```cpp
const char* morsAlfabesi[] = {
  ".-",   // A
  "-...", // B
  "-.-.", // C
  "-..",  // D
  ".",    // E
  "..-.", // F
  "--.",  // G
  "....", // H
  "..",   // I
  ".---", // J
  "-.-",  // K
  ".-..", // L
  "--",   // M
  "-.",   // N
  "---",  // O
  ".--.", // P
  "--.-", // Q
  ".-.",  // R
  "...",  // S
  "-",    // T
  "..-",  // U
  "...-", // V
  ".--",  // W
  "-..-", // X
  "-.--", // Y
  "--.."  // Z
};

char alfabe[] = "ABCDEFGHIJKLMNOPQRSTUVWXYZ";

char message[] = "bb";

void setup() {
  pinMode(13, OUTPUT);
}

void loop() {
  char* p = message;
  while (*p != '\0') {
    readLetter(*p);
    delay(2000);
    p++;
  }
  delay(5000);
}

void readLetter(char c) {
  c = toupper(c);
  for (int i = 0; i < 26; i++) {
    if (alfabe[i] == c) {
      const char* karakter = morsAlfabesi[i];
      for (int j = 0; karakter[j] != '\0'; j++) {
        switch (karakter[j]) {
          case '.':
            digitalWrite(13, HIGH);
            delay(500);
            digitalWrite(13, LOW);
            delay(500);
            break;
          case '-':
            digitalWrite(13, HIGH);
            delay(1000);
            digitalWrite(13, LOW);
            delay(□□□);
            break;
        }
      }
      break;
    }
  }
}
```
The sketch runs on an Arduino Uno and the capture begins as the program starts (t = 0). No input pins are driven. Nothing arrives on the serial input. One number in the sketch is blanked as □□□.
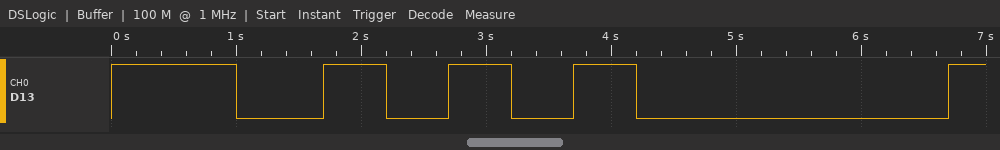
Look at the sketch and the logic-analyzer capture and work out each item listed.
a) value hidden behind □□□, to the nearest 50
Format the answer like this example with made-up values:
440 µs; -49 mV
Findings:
700
